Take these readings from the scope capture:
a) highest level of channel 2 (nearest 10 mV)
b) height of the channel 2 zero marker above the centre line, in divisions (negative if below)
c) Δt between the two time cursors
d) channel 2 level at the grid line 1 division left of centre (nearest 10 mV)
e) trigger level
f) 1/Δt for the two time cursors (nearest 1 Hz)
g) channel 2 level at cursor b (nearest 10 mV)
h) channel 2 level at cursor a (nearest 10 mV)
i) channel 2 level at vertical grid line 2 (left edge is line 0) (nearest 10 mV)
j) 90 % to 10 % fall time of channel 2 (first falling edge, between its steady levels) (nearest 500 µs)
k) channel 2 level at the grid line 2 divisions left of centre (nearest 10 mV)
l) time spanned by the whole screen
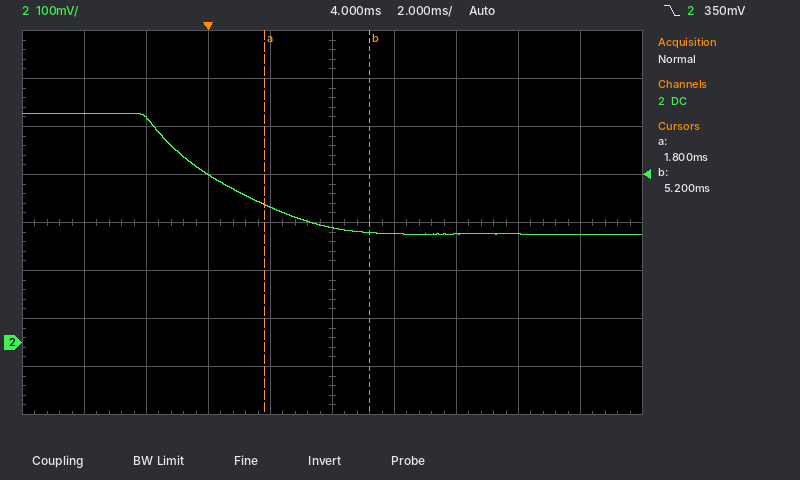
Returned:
480 mV
-2.5 div
3.4 ms
280 mV
350 mV
294 Hz
230 mV
290 mV
470 mV
5.0 ms
350 mV
20 ms
